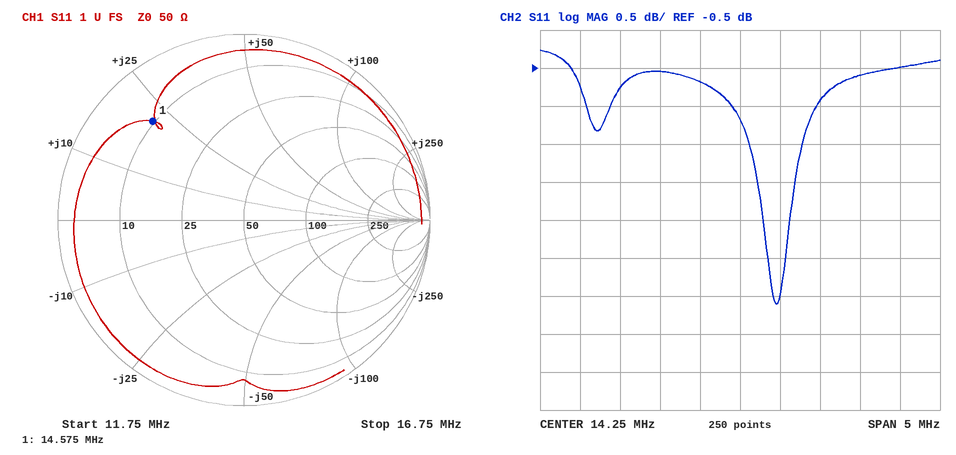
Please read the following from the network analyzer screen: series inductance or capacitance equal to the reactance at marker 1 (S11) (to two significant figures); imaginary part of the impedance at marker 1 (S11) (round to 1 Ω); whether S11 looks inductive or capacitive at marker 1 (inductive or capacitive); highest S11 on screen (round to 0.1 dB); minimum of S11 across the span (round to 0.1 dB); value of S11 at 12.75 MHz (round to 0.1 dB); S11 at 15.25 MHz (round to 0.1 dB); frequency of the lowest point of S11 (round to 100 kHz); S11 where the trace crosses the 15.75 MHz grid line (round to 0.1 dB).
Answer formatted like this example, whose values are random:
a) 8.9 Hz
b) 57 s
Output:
a) 230 nH
b) +21 Ω
c) inductive
d) -0.3 dB
e) -3.6 dB
f) -0.8 dB
g) -0.9 dB
h) 14.7 MHz
i) -0.6 dB
